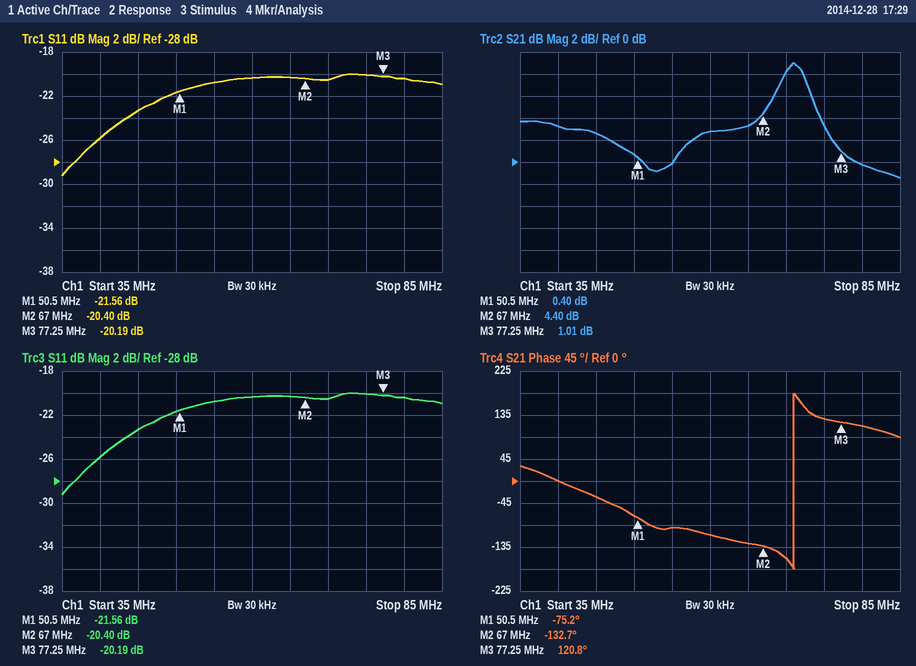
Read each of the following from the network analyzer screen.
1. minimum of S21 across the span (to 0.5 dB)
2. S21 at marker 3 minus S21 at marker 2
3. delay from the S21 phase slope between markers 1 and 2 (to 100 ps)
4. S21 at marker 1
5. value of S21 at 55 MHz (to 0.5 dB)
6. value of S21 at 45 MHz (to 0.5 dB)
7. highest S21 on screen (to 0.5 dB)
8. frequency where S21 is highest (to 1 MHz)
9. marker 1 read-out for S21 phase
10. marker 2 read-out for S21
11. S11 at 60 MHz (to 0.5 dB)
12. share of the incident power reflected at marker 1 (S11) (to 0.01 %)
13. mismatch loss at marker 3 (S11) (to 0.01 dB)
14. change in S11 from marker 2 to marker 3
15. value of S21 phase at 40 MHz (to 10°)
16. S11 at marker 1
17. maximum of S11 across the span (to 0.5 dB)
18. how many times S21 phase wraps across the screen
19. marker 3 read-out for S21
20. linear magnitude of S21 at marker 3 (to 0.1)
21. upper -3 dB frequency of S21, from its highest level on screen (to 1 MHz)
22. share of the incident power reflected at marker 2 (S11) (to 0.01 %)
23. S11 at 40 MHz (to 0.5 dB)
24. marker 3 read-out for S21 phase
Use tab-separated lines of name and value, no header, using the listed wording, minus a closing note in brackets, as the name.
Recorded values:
minimum of S21 across the span	-1.5 dB
S21 at marker 3 minus S21 at marker 2	-3.39 dB
delay from the S21 phase slope between markers 1 and 2	9.7 ns
S21 at marker 1	0.40 dB
value of S21 at 55 MHz	0.0 dB
value of S21 at 45 MHz	2.5 dB
highest S21 on screen	9.0 dB
frequency where S21 is highest	71 MHz
marker 1 read-out for S21 phase	-75.2°
marker 2 read-out for S21	4.40 dB
S11 at 60 MHz	-20.5 dB
share of the incident power reflected at marker 1 (S11)	0.70 %
mismatch loss at marker 3 (S11)	0.04 dB
change in S11 from marker 2 to marker 3	0.21 dB
value of S21 phase at 40 MHz	0°
S11 at marker 1	-21.56 dB
maximum of S11 across the span	-20.0 dB
how many times S21 phase wraps across the screen	1
marker 3 read-out for S21	1.01 dB
linear magnitude of S21 at marker 3	1.1
upper -3 dB frequency of S21, from its highest level on screen	73 MHz
share of the incident power reflected at marker 2 (S11)	0.91 %
S11 at 40 MHz	-26.0 dB
marker 3 read-out for S21 phase	120.8°
